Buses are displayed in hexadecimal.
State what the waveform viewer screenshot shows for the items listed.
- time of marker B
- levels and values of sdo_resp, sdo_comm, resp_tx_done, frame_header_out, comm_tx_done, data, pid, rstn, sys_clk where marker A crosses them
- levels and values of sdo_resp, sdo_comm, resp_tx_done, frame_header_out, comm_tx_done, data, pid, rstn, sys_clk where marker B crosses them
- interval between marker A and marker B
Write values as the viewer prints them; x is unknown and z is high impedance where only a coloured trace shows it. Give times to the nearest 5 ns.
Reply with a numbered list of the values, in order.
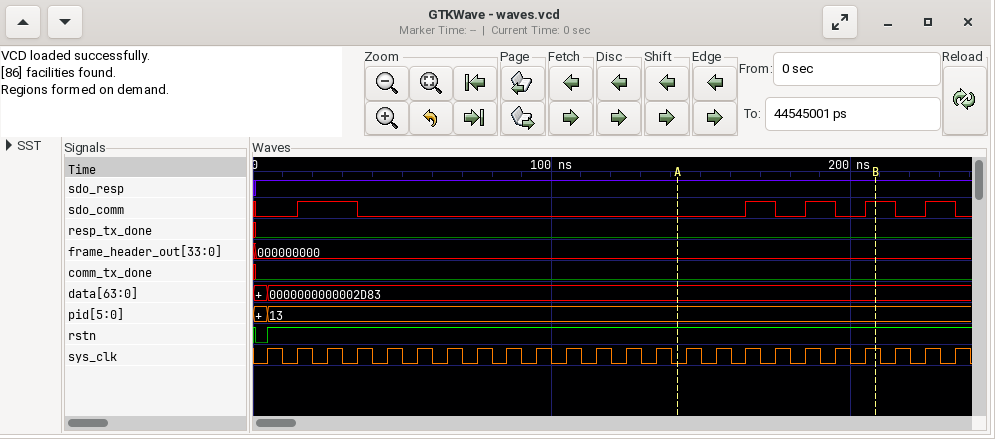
1. 210 ns
2. sdo_resp=1, sdo_comm=0, resp_tx_done=0, frame_header_out=000000000, comm_tx_done=0, data=0000000000002D83, pid=13, rstn=1, sys_clk=0
3. sdo_resp=1, sdo_comm=1, resp_tx_done=0, frame_header_out=000000000, comm_tx_done=0, data=0000000000002D83, pid=13, rstn=1, sys_clk=1
4. 65 ns
